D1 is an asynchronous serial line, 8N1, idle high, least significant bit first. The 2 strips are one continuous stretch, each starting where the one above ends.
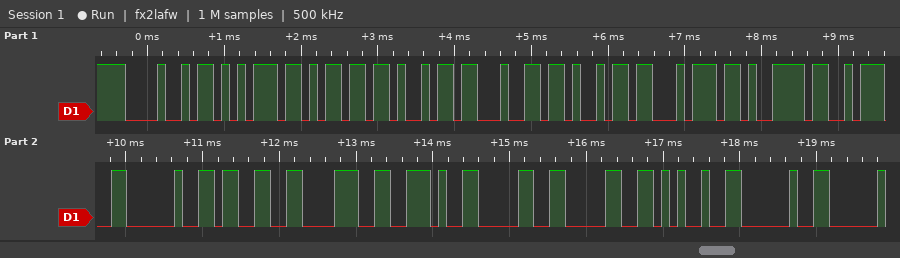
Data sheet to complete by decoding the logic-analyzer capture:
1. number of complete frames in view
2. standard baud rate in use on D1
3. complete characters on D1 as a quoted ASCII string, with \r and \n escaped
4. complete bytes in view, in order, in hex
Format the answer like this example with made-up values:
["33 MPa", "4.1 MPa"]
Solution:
["17", "9600 baud", "\"Humidity: 38.00% \"", "0x48 0x75 0x6D 0x69 0x64 0x69 0x74 0x79 0x3A 0x20 0x33 0x38 0x2E 0x30 0x30 0x25 0x20"]
